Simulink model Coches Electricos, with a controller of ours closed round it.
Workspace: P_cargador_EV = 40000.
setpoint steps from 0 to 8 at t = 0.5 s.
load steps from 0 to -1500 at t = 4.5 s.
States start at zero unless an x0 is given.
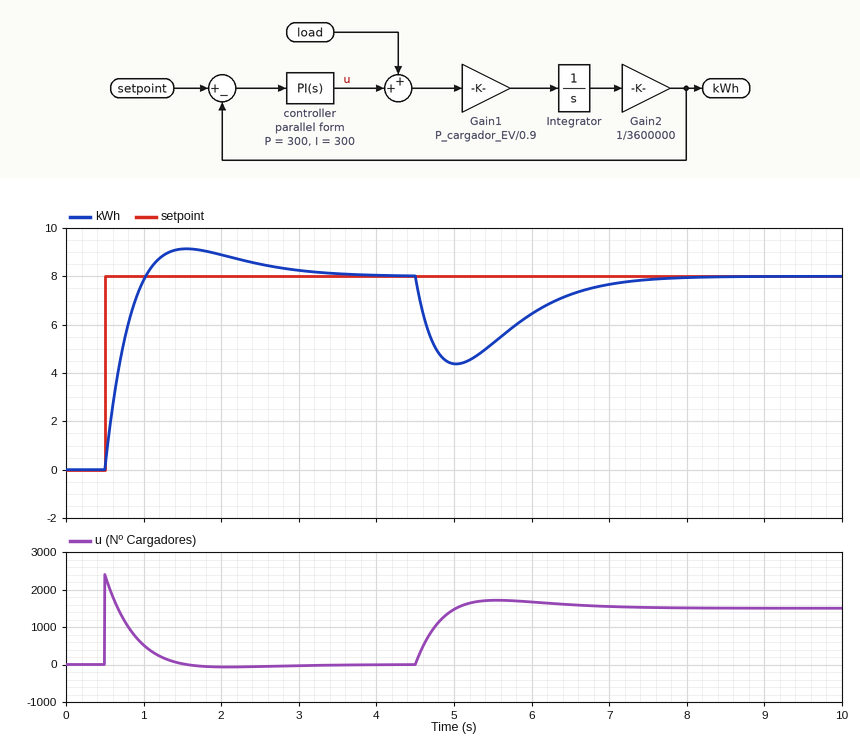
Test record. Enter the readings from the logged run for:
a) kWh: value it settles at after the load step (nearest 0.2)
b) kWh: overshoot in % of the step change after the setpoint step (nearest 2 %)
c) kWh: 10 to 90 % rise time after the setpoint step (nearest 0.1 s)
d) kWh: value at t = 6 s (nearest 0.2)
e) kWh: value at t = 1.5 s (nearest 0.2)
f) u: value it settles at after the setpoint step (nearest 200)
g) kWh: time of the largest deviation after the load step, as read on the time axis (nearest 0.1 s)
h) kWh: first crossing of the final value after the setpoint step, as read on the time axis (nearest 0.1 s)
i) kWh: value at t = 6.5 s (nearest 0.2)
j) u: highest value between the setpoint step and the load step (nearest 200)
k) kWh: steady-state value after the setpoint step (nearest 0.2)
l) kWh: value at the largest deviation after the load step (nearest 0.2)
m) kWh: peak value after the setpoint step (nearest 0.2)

8.0
14 %
0.4 s
6.4
9.2
0
5.0 s
1.0 s
7.2
2400
8.0
4.4
9.2
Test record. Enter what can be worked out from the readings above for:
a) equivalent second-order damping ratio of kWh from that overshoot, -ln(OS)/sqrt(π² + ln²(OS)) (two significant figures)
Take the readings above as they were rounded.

0.53
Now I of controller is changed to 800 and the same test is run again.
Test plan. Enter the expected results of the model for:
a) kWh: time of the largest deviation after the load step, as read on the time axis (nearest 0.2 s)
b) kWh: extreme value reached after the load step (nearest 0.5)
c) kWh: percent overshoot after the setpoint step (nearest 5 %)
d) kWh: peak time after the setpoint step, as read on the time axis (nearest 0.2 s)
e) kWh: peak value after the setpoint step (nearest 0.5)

4.8 s
5.0
25 %
1.2 s
10.0
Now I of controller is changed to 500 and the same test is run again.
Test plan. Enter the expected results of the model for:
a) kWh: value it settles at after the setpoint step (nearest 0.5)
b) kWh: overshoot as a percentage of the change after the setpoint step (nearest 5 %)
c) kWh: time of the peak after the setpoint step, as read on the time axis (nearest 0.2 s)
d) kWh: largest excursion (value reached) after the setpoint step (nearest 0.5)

8.0
20 %
1.4 s
9.5
